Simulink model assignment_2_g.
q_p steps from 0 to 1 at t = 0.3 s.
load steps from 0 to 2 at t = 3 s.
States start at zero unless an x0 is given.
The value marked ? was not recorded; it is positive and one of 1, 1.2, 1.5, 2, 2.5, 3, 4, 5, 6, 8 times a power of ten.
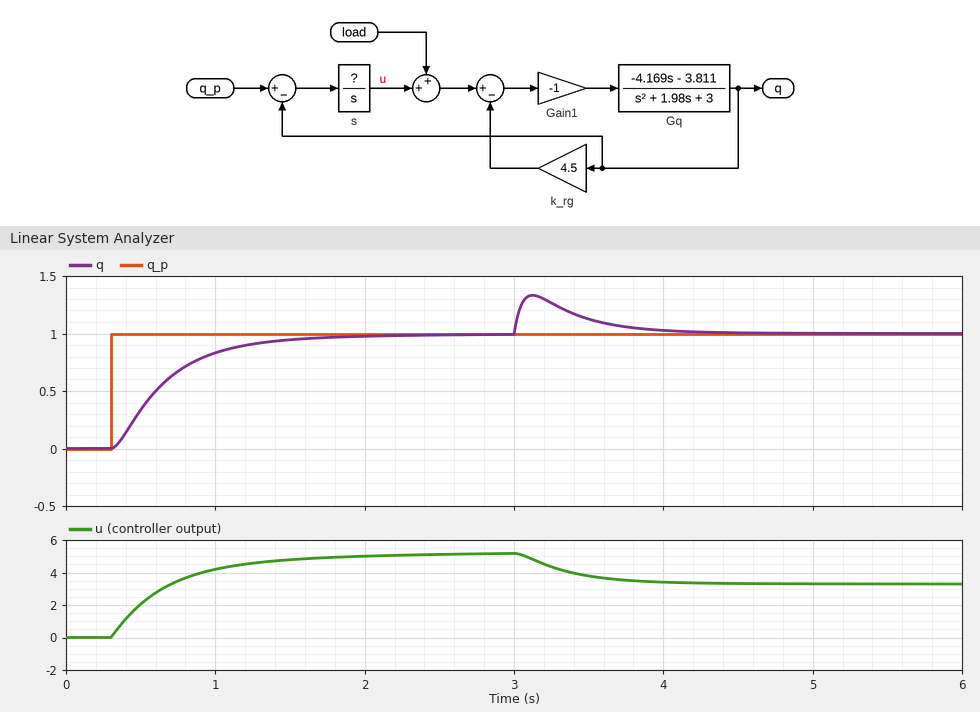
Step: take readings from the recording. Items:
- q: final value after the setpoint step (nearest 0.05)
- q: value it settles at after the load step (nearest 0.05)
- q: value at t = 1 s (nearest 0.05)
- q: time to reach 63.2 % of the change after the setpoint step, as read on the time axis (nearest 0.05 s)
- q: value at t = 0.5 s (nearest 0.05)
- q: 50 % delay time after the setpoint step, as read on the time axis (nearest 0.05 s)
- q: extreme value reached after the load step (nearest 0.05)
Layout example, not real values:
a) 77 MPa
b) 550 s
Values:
a) 1.00
b) 1.00
c) 0.85
d) 0.70 s
e) 0.35
f) 0.60 s
g) 1.35
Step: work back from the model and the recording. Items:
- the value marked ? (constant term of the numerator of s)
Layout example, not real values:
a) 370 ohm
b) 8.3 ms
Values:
a) 12
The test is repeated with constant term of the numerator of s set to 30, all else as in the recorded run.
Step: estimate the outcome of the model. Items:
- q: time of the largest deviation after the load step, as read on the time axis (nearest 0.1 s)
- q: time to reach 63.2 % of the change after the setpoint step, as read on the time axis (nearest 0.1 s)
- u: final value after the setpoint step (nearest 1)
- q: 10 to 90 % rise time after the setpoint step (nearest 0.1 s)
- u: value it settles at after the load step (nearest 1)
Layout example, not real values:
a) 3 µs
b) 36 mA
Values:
a) 3.1 s
b) 0.5 s
c) 5
d) 0.3 s
e) 3
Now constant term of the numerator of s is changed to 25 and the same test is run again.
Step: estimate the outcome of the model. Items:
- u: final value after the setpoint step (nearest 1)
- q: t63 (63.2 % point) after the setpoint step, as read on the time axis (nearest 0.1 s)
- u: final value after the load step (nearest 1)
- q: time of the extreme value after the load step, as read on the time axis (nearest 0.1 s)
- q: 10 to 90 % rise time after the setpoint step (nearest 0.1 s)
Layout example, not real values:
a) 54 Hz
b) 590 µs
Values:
a) 5
b) 0.5 s
c) 3
d) 3.1 s
e) 0.3 s
